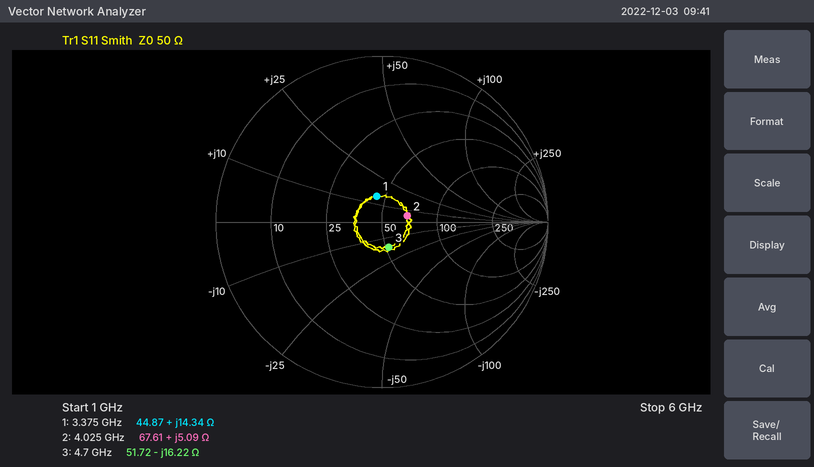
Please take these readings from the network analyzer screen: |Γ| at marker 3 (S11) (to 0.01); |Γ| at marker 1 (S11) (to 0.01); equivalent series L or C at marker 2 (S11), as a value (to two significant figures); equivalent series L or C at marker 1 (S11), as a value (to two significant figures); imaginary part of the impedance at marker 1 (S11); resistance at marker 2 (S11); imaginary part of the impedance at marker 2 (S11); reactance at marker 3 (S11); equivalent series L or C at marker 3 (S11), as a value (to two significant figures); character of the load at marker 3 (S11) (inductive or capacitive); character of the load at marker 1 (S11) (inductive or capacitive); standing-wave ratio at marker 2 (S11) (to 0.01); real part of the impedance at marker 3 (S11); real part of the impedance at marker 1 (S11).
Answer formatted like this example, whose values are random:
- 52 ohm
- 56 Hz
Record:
- 0.16
- 0.16
- 200 pH
- 680 pH
- +14.34 Ω
- 67.61 Ω
- +5.09 Ω
- -16.22 Ω
- 2.1 pF
- capacitive
- inductive
- 1.37
- 51.72 Ω
- 44.87 Ω
